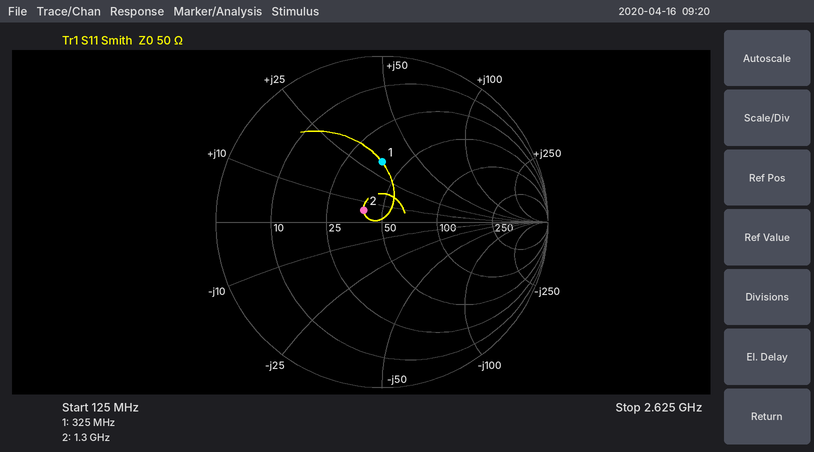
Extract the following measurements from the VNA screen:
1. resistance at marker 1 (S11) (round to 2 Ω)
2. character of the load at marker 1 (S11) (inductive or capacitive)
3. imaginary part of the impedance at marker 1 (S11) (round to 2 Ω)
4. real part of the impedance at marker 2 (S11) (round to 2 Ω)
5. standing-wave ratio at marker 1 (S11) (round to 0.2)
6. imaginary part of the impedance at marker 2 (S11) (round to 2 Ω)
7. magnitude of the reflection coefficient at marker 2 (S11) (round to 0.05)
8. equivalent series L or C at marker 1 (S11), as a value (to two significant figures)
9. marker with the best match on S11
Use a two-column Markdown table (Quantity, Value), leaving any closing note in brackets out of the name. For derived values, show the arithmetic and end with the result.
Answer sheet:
| Quantity | Value |
|---|---|
| resistance at marker 1 (S11) | 38 Ω |
| character of the load at marker 1 (S11) | inductive |
| imaginary part of the impedance at marker 1 (S11) | +32 Ω |
| real part of the impedance at marker 2 (S11) | 40 Ω |
| standing-wave ratio at marker 1 (S11) | 2.2 |
| imaginary part of the impedance at marker 2 (S11) | +6 Ω |
| magnitude of the reflection coefficient at marker 2 (S11) | 0.15 |
| equivalent series L or C at marker 1 (S11), as a value | L = 32 Ω/(2π × 325 MHz) ≈ 16 nH |
| marker with the best match on S11 | marker 2 |
